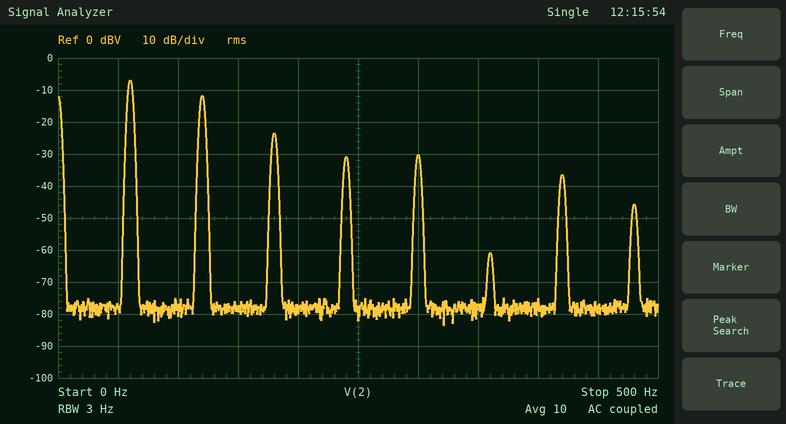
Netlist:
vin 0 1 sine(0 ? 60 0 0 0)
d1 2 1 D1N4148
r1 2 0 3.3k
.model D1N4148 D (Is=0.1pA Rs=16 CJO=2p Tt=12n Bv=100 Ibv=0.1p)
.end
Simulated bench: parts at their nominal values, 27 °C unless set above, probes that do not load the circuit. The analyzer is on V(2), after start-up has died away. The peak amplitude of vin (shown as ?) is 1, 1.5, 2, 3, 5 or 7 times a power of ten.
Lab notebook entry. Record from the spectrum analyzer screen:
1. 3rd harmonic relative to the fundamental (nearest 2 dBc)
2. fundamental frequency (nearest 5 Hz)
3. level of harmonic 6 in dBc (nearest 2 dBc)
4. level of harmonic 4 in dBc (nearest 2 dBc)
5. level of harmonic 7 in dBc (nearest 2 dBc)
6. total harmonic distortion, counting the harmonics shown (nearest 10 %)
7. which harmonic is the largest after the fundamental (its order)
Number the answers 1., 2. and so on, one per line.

1. -16 dBc
2. 60 Hz
3. -54 dBc
4. -24 dBc
5. -30 dBc
6. 60 %
7. 2
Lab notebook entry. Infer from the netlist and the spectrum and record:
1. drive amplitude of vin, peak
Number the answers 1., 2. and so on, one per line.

1. 2 V
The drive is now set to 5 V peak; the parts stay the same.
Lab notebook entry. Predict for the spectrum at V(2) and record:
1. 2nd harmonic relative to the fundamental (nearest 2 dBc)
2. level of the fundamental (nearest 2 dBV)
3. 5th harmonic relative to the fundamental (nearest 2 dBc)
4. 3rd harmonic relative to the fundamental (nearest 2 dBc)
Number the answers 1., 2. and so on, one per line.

1. -6 dBc
2. 4 dBV
3. -30 dBc
4. -26 dBc
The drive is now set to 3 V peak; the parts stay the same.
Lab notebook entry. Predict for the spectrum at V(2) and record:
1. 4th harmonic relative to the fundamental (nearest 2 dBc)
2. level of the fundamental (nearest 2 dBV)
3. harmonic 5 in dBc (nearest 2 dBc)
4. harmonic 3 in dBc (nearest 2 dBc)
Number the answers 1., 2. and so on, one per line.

1. -22 dBc
2. -2 dBV
3. -26 dBc
4. -20 dBc
